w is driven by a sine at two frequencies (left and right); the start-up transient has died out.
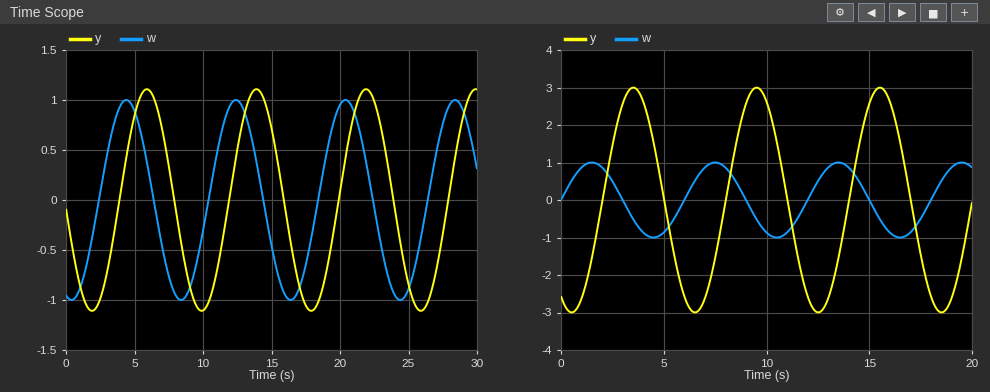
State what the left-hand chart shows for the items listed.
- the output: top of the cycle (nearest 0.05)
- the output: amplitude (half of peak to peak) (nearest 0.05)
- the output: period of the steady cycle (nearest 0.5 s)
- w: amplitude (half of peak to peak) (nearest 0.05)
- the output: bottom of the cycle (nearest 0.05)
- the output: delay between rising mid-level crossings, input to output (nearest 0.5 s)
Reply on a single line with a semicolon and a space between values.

1.10; 1.10; 8.0 s; 1.00; -1.10; 1.5 s
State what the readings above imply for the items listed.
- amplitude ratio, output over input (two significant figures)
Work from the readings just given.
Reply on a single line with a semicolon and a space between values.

1.1
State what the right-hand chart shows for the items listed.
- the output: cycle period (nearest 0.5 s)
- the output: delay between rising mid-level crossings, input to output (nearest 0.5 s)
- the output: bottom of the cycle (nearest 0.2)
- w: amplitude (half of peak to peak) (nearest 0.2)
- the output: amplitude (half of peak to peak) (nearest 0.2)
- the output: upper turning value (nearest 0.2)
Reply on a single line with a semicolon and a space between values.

6.0 s; 2.0 s; -3.0; 1.0; 3.0; 3.0
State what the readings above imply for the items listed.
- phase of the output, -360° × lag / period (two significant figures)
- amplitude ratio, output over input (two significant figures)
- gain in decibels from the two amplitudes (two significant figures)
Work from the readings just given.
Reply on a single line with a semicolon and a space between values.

-120°; 3.0; 9.5 dB
